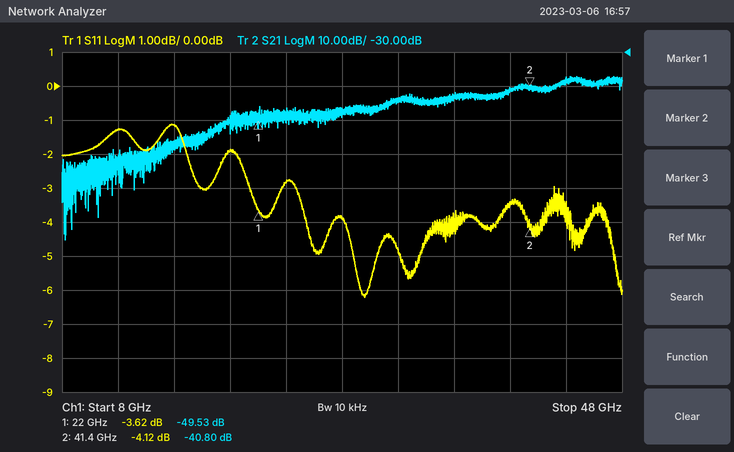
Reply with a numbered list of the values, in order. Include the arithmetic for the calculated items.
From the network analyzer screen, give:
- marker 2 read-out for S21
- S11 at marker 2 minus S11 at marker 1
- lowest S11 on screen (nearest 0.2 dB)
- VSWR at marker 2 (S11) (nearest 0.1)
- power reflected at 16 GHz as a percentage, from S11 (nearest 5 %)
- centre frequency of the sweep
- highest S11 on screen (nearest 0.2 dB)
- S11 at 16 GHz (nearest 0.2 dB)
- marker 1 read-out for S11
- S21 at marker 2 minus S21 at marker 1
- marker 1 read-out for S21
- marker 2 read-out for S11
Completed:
1. -40.80 dB
2. -4.12 − (-3.62) = -0.50 dB
3. -6.2 dB
4. (1 + 0.6223)/(1 − 0.6223) ≈ 4.3
5. 10^(-1.2/10) ≈ 75.9 %, so 75 % to the nearest 5 %
6. 28 GHz
7. -1.2 dB
8. -1.2 dB
9. -3.62 dB
10. -40.8 − (-49.53) = 8.73 dB
11. -49.53 dB
12. -4.12 dB
